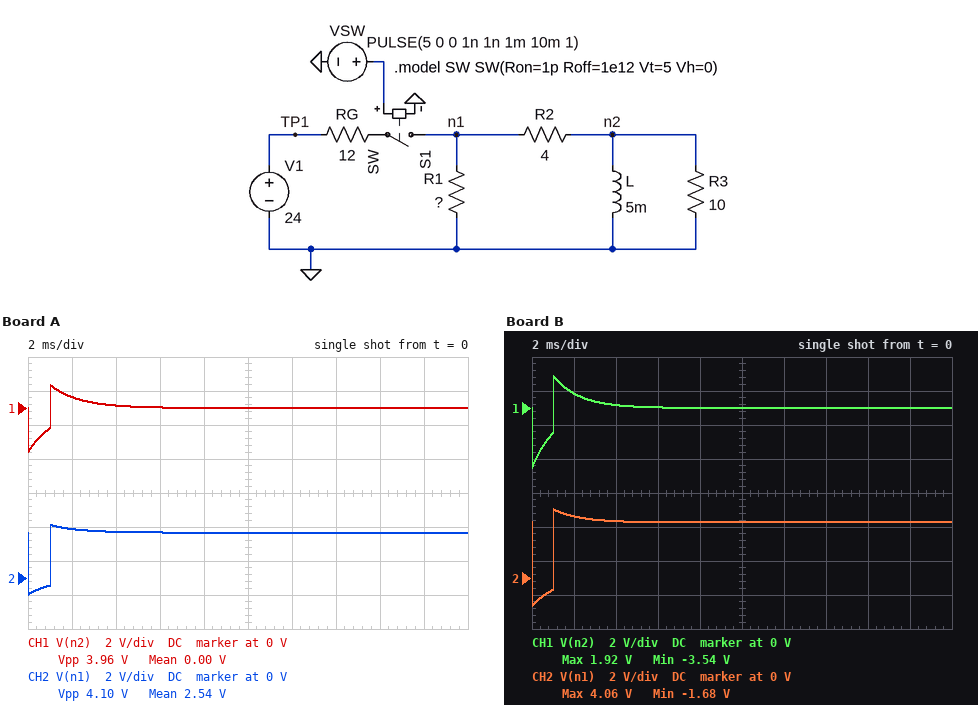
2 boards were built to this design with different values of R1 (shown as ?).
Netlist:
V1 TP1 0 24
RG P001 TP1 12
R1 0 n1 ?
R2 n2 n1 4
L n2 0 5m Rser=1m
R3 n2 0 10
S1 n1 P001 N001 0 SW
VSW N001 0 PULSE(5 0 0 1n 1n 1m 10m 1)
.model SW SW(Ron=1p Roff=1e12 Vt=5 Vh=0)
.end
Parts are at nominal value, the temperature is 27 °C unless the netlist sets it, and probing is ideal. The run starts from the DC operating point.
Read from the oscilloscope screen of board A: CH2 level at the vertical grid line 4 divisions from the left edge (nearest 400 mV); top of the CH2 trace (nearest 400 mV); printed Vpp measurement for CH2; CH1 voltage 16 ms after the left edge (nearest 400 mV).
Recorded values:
2.8 V
3.2 V
4.10 V
0 V
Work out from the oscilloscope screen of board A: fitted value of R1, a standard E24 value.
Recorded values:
2.4 Ω
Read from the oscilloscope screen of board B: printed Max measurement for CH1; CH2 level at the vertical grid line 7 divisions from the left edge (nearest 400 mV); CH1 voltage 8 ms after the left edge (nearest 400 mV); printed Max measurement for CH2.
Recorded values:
1.92 V
3.2 V
0 V
4.06 V
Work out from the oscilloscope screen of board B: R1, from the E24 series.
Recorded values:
3.6 Ω
